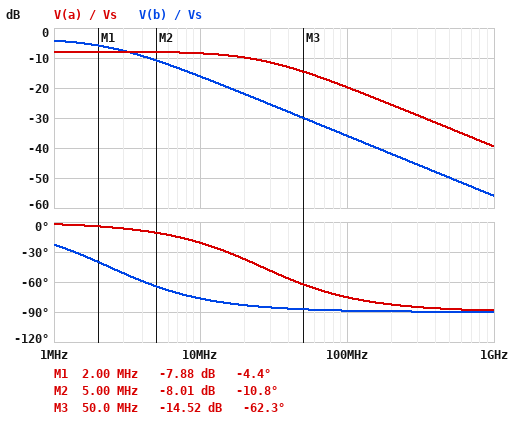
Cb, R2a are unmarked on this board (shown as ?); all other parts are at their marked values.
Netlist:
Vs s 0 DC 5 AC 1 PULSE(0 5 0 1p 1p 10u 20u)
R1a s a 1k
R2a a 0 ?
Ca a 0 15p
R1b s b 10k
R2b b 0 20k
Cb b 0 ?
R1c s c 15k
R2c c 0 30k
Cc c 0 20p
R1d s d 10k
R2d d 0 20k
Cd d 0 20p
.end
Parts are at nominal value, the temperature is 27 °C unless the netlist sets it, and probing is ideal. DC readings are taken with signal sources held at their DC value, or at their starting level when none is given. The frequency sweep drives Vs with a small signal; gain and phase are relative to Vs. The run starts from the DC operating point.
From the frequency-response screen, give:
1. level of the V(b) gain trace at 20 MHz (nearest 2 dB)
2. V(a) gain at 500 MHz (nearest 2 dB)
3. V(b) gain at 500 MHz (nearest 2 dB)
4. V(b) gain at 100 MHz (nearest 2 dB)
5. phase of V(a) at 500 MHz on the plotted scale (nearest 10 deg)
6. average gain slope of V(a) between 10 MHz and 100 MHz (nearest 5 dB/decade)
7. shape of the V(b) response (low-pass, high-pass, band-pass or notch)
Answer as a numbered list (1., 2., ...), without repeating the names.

1. -22 dB
2. -34 dB
3. -50 dB
4. -36 dB
5. -90 deg
6. -10 dB/decade
7. low-pass
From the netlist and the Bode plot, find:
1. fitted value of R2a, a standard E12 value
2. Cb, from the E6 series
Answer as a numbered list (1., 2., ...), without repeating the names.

1. 680 Ω
2. 10 pF
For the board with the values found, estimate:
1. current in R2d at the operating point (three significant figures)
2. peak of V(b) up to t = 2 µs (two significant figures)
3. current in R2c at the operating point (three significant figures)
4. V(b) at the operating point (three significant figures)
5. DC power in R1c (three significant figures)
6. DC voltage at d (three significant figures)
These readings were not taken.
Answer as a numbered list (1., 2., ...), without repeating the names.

1. 167 µA
2. 3.3 V
3. 111 µA
4. 3.33 V
5. 185 µW
6. 3.33 V
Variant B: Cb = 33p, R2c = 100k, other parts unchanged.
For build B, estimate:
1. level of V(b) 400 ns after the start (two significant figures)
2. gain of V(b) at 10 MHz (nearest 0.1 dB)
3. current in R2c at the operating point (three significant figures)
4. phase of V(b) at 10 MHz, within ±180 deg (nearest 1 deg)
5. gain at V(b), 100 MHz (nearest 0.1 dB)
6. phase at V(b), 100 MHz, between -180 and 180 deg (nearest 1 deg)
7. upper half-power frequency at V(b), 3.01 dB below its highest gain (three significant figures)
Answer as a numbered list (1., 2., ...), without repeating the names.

1. 2.8 V
2. -26.4 dB
3. 43.5 µA
4. -86 deg
5. -46.3 dB
6. -90 deg
7. 723 kHz
